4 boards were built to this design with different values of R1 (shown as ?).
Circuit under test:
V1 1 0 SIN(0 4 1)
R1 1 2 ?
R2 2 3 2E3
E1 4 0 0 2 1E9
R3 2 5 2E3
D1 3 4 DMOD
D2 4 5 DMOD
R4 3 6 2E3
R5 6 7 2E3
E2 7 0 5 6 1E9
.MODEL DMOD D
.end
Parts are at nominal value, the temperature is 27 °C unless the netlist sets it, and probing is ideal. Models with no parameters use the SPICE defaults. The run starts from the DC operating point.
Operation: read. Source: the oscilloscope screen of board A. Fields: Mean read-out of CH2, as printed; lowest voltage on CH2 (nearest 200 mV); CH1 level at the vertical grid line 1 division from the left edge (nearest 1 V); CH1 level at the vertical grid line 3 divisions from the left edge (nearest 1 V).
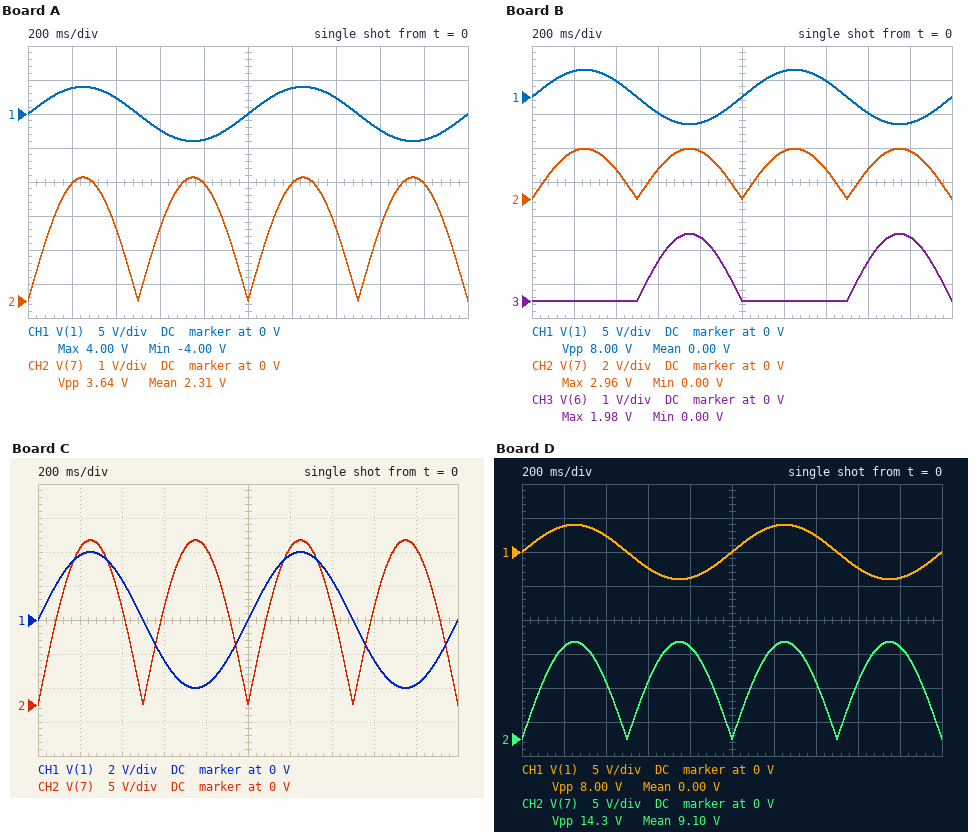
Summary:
2.31 V
0 V
4 V
-2 V
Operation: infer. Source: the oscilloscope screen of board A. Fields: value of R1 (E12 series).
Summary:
2.2 kΩ
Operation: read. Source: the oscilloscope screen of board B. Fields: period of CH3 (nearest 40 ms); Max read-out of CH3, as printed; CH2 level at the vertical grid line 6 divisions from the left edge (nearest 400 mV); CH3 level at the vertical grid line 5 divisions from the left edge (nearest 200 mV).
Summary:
1.00 s
1.98 V
2.8 V
0 V
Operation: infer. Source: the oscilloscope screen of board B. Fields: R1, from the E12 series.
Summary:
2.7 kΩ
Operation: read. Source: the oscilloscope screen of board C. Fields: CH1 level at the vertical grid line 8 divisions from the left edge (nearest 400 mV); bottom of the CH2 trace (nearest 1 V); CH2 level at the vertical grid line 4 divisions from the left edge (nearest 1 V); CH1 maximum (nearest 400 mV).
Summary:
-2.4 V
0 V
23 V
4.0 V
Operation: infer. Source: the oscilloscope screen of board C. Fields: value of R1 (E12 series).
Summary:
330 Ω
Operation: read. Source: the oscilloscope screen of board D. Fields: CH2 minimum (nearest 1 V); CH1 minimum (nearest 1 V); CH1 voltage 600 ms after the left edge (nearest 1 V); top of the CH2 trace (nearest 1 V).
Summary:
0 V
-4 V
-2 V
14 V
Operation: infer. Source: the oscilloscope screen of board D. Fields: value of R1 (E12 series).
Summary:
560 Ω
